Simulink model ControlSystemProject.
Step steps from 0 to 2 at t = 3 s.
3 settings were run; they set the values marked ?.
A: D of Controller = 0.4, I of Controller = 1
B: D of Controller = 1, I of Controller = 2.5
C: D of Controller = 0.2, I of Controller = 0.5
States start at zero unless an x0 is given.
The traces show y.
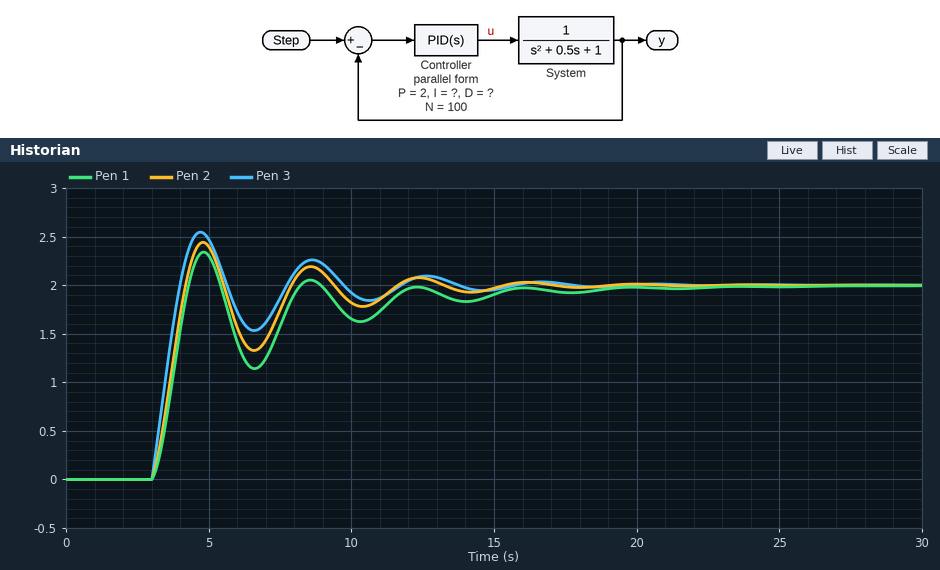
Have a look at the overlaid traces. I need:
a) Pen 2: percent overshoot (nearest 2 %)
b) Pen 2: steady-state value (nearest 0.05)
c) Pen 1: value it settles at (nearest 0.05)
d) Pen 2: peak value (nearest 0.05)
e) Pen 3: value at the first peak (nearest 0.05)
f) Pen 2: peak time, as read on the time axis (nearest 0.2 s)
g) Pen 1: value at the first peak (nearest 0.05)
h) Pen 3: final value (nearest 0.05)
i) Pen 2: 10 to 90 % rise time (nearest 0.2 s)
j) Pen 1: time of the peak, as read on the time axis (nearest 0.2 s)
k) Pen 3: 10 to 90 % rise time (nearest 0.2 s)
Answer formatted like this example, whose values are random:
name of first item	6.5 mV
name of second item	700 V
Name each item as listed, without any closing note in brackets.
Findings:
Pen 2: percent overshoot	22 %
Pen 2: steady-state value	2.00
Pen 1: value it settles at	2.00
Pen 2: peak value	2.45
Pen 3: value at the first peak	2.55
Pen 2: peak time, as read on the time axis	4.8 s
Pen 1: value at the first peak	2.35
Pen 3: final value	2.00
Pen 2: 10 to 90 % rise time	0.8 s
Pen 1: time of the peak, as read on the time axis	4.8 s
Pen 3: 10 to 90 % rise time	0.8 s
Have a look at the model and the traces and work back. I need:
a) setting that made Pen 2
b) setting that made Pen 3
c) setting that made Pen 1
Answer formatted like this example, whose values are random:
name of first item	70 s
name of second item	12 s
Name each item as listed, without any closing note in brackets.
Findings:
setting that made Pen 2	A
setting that made Pen 3	B
setting that made Pen 1	C
